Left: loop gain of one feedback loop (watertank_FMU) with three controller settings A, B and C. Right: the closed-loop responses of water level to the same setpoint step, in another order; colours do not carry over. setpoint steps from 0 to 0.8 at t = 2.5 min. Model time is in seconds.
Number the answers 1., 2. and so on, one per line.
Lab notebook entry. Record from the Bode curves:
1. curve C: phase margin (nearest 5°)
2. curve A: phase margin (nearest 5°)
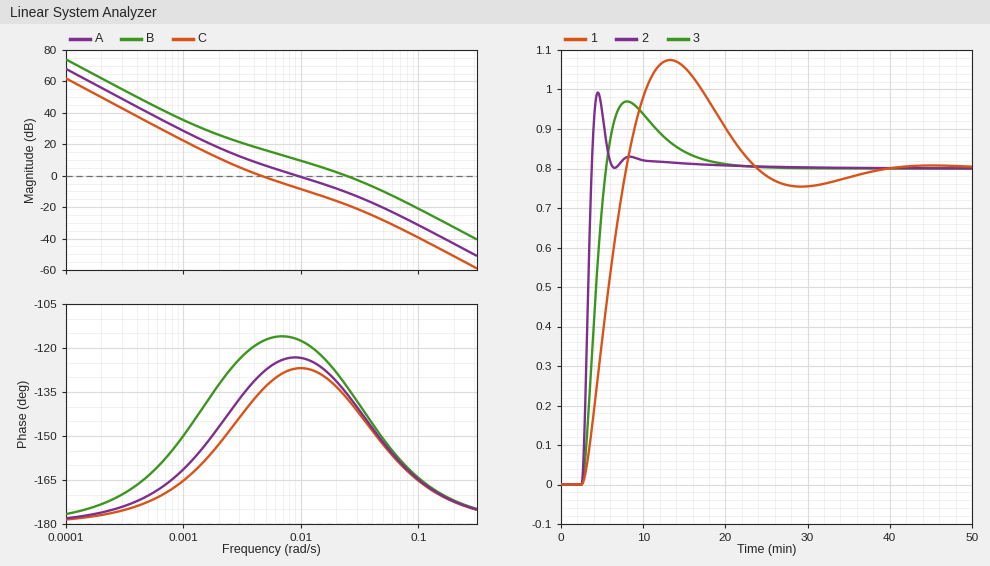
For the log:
1. 45°
2. 55°
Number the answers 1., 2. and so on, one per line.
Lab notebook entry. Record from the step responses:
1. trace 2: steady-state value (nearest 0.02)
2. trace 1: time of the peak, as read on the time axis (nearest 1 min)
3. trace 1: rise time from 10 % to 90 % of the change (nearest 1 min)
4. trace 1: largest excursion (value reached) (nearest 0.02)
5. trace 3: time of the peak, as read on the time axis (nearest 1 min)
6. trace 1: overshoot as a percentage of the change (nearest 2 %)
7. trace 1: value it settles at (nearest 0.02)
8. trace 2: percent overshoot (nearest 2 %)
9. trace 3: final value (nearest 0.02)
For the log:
1. 0.80
2. 13 min
3. 4 min
4. 1.08
5. 8 min
6. 34 %
7. 0.80
8. 24 %
9. 0.80
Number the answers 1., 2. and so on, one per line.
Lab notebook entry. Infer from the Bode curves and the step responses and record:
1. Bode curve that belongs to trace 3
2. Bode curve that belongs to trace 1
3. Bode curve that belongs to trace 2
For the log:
1. A
2. C
3. B
